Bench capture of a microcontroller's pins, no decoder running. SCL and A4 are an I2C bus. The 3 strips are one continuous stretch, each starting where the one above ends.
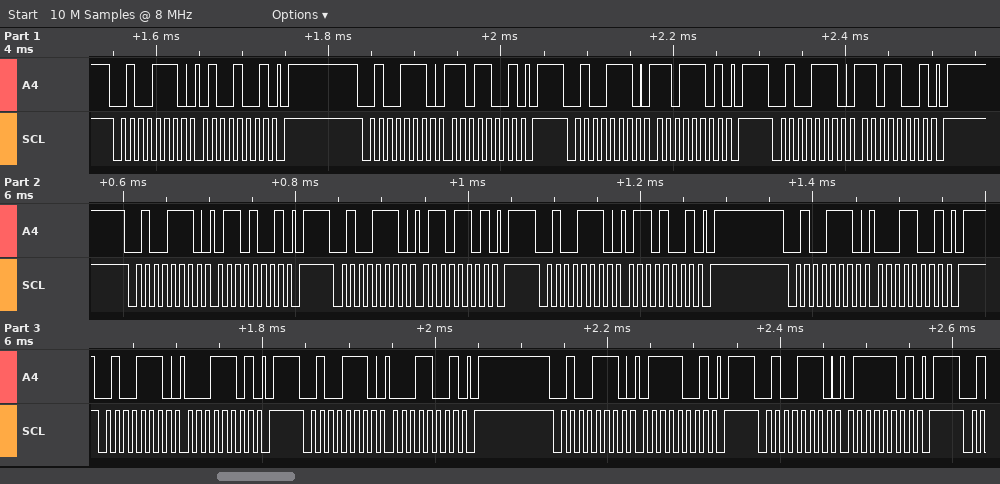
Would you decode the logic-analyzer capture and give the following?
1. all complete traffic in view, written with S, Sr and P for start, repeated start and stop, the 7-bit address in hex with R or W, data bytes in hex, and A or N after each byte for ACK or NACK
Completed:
S 27W A 49 A P S 27W A D9 A P S 27W A DD A P S 27W A D9 A P S 27W A 69 A P S 27W A 6D A P S 27W A 69 A P S 27W A 19 A P S 27W A 1D A P S 27W A 19 A P S 27W A 79 A P S 27W A 7D A P
